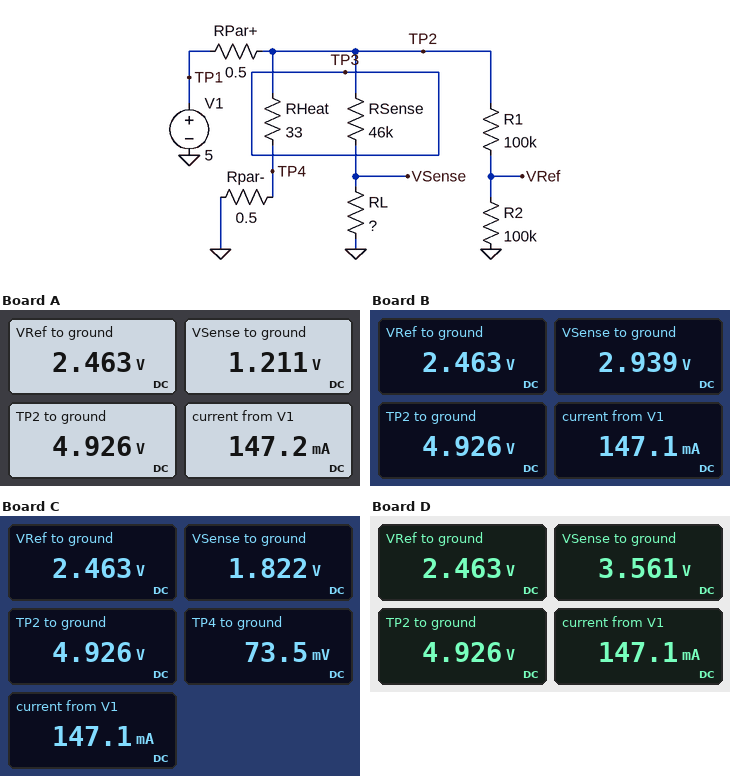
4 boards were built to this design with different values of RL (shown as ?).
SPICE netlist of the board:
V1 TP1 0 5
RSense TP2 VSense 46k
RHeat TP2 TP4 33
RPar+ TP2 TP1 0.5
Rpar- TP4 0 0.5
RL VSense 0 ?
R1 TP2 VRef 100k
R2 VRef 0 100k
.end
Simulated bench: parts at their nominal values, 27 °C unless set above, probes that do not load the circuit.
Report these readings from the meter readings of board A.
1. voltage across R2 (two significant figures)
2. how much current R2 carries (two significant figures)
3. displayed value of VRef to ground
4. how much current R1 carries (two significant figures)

2.5 V
25 µA
2.463 V
25 µA
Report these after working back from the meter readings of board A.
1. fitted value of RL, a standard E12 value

15 kΩ
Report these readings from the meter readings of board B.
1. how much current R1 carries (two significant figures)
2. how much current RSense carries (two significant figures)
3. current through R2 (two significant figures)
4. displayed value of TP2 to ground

25 µA
43 µA
25 µA
4.926 V
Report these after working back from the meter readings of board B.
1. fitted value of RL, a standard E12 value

68 kΩ
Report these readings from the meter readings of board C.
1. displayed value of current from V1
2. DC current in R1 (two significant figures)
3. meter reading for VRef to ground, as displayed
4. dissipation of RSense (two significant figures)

147.1 mA
25 µA
2.463 V
210 µW
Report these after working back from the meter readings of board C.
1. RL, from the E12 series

27 kΩ
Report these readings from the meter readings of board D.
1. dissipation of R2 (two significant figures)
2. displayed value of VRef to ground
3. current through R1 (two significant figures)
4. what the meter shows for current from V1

61 µW
2.463 V
25 µA
147.1 mA
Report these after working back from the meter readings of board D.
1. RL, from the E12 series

120 kΩ
